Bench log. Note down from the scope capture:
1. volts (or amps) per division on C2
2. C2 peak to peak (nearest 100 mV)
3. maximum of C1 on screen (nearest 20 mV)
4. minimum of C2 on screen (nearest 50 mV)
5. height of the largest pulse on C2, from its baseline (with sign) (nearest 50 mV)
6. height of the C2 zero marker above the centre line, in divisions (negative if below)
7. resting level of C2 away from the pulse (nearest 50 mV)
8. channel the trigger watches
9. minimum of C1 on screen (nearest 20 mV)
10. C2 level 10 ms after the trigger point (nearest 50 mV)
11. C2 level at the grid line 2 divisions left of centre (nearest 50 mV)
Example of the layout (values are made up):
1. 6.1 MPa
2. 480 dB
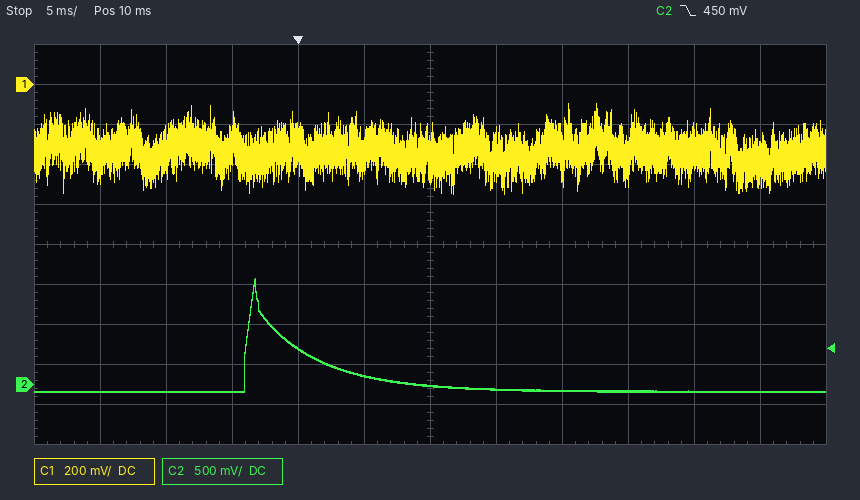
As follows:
1. 500 mV
2. 1.40 V
3. -100 mV
4. -100 mV
5. +1.40 V
6. -3.5 div
7. -100 mV
8. C2
9. -540 mV
10. 0 mV
11. 450 mV
